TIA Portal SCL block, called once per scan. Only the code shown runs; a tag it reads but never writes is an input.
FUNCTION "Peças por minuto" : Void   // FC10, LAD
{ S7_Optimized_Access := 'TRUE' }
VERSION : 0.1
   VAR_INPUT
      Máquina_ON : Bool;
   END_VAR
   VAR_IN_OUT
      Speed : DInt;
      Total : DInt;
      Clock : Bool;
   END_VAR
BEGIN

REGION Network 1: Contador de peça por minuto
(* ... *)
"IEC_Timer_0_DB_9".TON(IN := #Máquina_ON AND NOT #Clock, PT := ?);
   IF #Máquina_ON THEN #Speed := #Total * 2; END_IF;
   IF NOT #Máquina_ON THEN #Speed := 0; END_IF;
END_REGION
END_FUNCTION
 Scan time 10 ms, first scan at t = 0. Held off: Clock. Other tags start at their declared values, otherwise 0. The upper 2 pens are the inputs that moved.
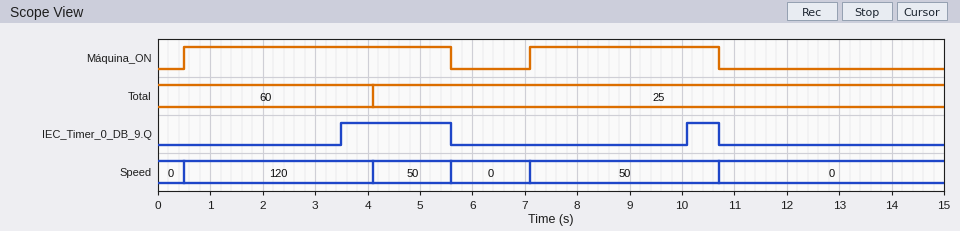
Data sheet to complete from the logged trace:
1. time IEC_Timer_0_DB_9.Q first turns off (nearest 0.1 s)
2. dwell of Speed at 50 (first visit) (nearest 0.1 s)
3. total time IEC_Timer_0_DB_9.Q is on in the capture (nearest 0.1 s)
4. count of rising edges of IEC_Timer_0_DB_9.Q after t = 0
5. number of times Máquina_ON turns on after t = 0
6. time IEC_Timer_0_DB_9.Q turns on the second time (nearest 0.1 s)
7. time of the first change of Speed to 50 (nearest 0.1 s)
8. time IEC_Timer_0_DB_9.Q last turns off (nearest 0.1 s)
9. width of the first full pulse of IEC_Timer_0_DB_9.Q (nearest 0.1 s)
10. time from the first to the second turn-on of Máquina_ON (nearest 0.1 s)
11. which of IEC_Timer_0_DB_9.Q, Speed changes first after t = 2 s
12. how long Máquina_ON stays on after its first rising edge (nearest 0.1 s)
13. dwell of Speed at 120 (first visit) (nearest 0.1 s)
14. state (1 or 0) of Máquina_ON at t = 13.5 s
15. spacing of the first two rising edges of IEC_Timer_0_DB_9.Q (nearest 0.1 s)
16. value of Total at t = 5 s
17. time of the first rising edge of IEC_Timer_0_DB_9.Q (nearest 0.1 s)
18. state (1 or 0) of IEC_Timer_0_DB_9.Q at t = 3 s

5.6 s
1.5 s
2.7 s
2
2
10.1 s
4.1 s
10.7 s
2.1 s
6.6 s
IEC_Timer_0_DB_9.Q
5.1 s
3.6 s
0
6.6 s
25
3.5 s
0
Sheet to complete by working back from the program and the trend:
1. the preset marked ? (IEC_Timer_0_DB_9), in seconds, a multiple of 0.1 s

3.0 s
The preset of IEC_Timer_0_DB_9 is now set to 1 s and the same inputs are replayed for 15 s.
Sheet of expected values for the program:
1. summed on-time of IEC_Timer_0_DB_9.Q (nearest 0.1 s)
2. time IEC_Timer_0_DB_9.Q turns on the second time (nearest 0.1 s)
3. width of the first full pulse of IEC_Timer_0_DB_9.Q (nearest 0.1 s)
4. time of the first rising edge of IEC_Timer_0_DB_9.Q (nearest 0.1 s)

6.7 s
8.1 s
4.1 s
1.5 s
